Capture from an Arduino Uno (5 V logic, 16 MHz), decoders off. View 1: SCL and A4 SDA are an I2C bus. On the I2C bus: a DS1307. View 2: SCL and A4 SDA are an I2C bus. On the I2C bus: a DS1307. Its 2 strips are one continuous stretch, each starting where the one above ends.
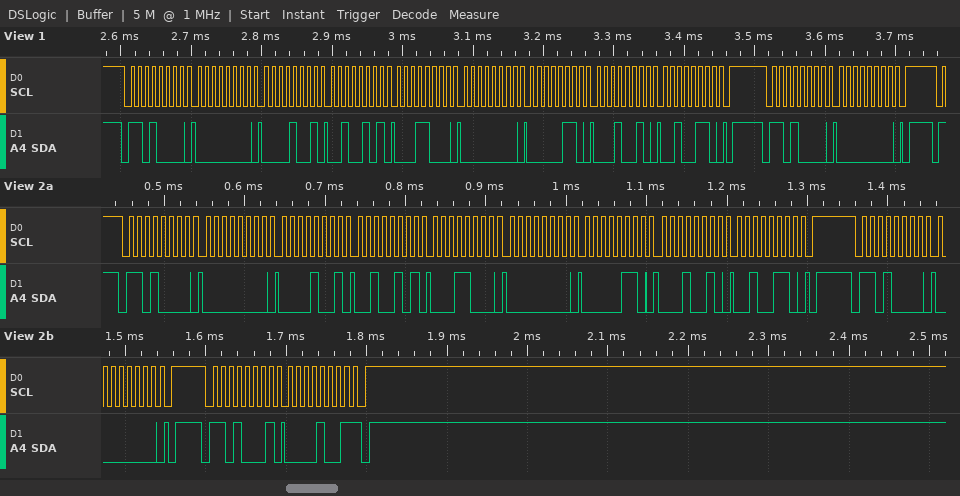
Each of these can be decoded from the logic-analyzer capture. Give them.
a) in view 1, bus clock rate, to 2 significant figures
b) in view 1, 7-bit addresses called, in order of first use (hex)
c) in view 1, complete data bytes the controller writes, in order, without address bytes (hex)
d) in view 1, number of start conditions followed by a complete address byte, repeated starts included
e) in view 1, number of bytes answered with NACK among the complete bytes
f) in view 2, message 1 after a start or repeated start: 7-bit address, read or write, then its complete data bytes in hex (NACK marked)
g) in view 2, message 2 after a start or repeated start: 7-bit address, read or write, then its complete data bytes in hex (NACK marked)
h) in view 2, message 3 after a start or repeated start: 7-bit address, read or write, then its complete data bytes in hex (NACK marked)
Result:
100 kHz
0x68
00 09 25 18 00 06 12 26 00
2
0
0x68 write: 00 09 25 18 00 06 12 26
0x68 write: 00
0x68 read: 09 NACK
